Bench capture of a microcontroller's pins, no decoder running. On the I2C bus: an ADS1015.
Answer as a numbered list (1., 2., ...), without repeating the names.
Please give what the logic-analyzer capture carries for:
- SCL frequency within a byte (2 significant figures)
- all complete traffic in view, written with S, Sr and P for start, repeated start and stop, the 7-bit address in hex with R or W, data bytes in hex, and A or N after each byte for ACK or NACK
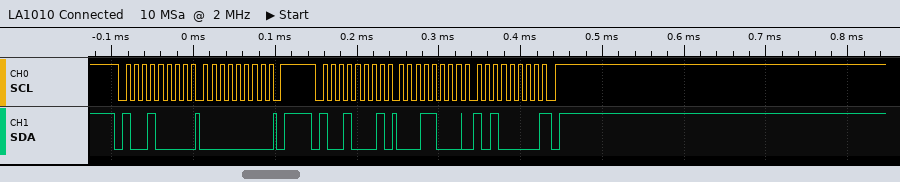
1. 100 kHz
2. S 48W A 00 A P S 48R A 18 A A0 N P
